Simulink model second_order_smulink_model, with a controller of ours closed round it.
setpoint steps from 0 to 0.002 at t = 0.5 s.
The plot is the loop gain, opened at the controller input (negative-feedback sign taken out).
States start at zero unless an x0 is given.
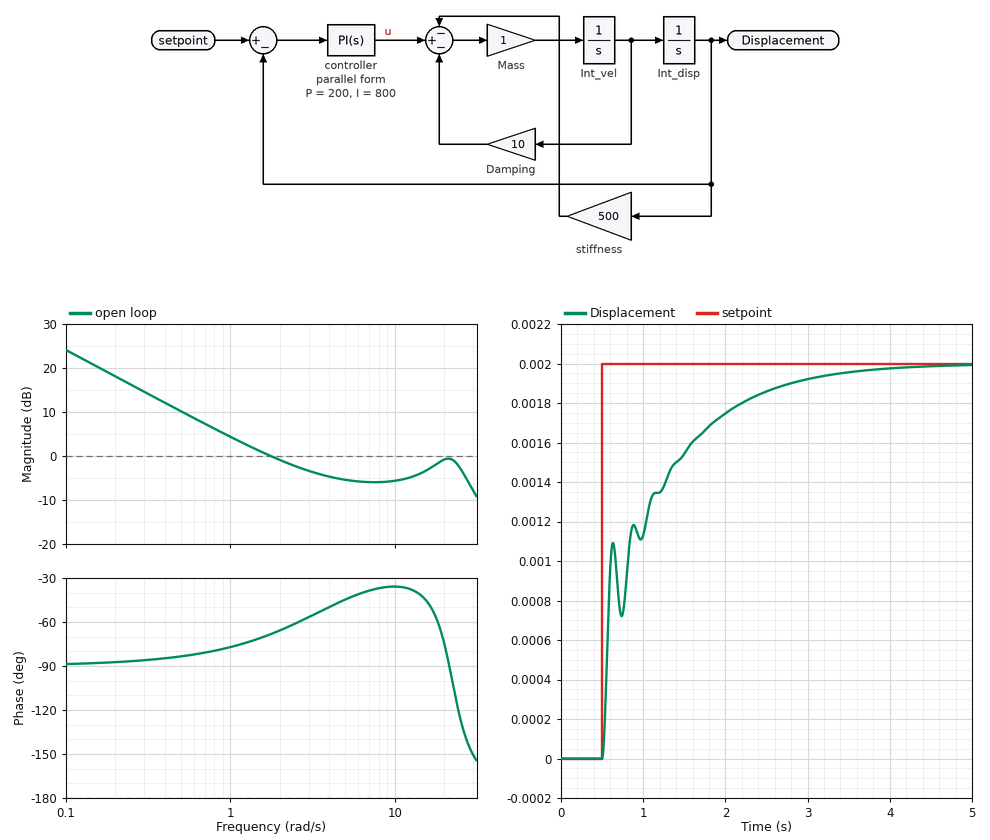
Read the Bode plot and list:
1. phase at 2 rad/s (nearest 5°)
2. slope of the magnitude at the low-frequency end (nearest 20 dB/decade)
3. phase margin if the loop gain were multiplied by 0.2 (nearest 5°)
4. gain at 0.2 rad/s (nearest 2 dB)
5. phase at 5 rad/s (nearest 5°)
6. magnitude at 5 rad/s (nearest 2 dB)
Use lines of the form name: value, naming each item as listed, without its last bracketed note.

phase at 2 rad/s: -65°
slope of the magnitude at the low-frequency end: -20 dB/decade
phase margin if the loop gain were multiplied by 0.2: 95°
gain at 0.2 rad/s: 18 dB
phase at 5 rad/s: -45°
magnitude at 5 rad/s: -6 dB
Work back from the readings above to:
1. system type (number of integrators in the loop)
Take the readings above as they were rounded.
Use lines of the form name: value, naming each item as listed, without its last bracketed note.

system type: 1
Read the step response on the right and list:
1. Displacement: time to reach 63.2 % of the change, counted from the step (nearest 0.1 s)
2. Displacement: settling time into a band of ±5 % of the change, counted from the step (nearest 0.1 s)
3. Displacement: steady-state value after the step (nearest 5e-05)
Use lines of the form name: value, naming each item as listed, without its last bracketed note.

Displacement: time to reach 63.2 % of the change, counted from the step: 0.6 s
Displacement: settling time into a band of ±5 % of the change, counted from the step: 2.3 s
Displacement: steady-state value after the step: 0.00200
